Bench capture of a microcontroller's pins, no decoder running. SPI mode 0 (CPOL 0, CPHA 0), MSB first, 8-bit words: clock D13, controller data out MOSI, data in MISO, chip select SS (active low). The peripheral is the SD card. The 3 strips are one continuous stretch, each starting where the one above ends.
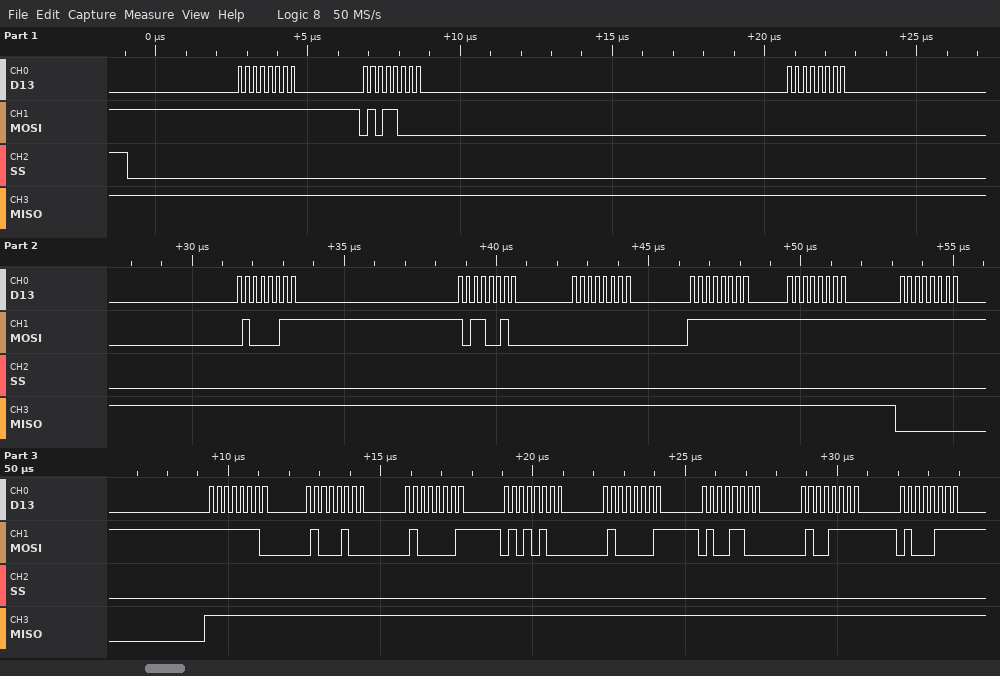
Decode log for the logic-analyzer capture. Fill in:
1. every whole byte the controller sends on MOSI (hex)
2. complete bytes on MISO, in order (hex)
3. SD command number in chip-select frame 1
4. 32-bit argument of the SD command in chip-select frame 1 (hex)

FF 58 00 43 B2 00 FF FF FF FE 44 41 54 41 4C 4F 47
FF FF FF FF FF FF FF FF 00 FF FF FF FF FF FF FF FF
CMD24
0x0043B200
